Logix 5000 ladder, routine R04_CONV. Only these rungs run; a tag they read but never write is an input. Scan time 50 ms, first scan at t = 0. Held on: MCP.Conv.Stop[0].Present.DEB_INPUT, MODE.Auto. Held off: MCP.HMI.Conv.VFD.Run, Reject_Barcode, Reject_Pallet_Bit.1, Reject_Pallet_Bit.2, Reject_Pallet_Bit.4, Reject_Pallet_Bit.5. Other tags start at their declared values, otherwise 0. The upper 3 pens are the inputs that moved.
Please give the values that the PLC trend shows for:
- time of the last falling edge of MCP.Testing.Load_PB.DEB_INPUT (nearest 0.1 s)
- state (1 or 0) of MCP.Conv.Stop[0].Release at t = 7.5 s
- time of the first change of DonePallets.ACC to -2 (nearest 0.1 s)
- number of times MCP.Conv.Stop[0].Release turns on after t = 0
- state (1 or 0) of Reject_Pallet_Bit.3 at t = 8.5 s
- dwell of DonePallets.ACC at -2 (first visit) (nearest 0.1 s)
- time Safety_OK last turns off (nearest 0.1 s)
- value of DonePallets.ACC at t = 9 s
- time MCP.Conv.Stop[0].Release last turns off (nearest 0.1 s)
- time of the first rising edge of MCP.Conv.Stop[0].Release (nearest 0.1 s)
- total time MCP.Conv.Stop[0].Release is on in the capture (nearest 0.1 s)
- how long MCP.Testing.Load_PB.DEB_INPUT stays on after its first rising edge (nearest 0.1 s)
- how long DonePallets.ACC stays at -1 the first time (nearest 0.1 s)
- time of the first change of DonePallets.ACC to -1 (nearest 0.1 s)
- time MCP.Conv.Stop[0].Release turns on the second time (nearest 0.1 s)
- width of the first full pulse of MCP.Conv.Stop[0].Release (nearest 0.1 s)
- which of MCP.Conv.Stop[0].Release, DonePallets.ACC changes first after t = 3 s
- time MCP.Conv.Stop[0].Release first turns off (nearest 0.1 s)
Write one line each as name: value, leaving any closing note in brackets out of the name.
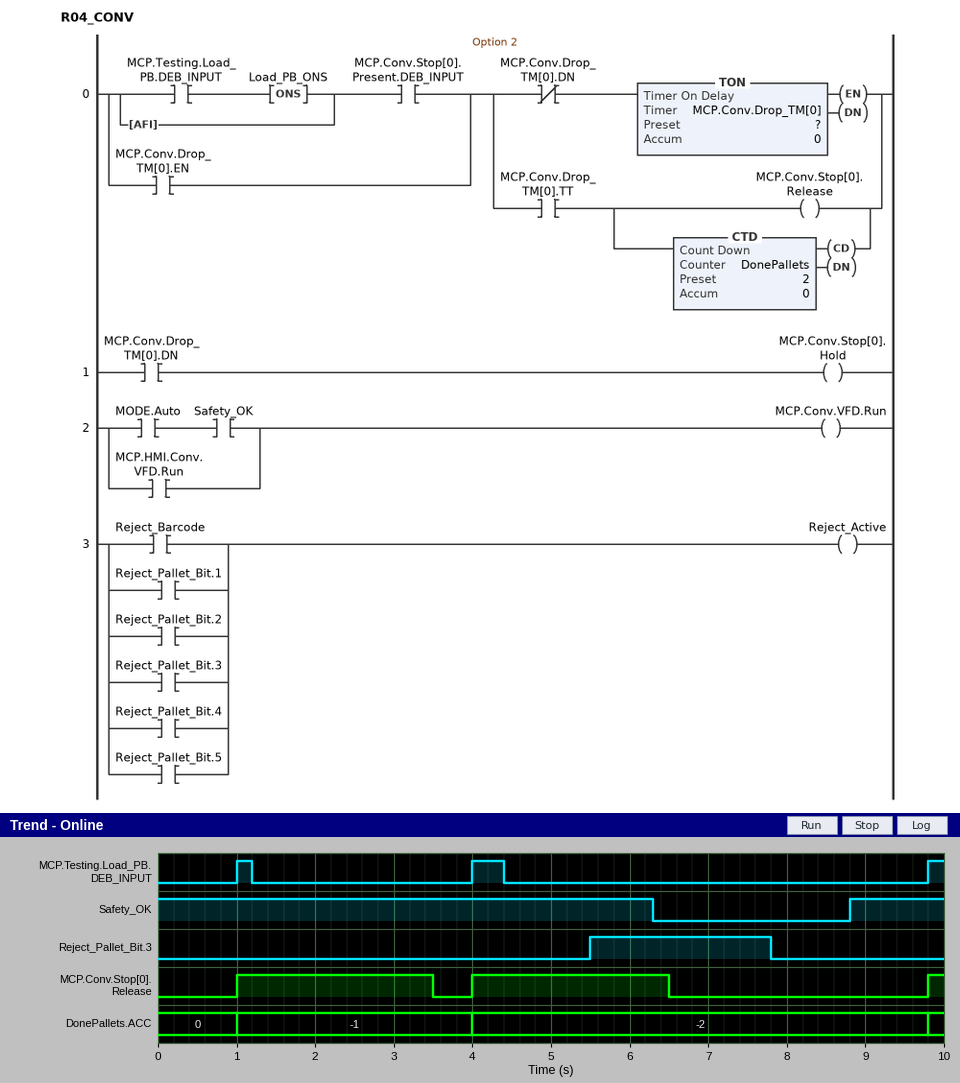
time of the last falling edge of MCP.Testing.Load_PB.DEB_INPUT: 4.4 s
state (1 or 0) of MCP.Conv.Stop[0].Release at t = 7.5 s: 0
time of the first change of DonePallets.ACC to -2: 4.0 s
number of times MCP.Conv.Stop[0].Release turns on after t = 0: 3
state (1 or 0) of Reject_Pallet_Bit.3 at t = 8.5 s: 0
dwell of DonePallets.ACC at -2 (first visit): 5.8 s
time Safety_OK last turns off: 6.3 s
value of DonePallets.ACC at t = 9 s: -2
time MCP.Conv.Stop[0].Release last turns off: 6.5 s
time of the first rising edge of MCP.Conv.Stop[0].Release: 1.0 s
total time MCP.Conv.Stop[0].Release is on in the capture: 5.2 s
how long MCP.Testing.Load_PB.DEB_INPUT stays on after its first rising edge: 0.2 s
how long DonePallets.ACC stays at -1 the first time: 3.0 s
time of the first change of DonePallets.ACC to -1: 1.0 s
time MCP.Conv.Stop[0].Release turns on the second time: 4.0 s
width of the first full pulse of MCP.Conv.Stop[0].Release: 2.5 s
which of MCP.Conv.Stop[0].Release, DonePallets.ACC changes first after t = 3 s: MCP.Conv.Stop[0].Release
time MCP.Conv.Stop[0].Release first turns off: 3.5 s
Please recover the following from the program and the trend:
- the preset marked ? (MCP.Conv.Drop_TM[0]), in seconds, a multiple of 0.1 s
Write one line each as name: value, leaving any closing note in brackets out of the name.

the preset marked ? (MCP.Conv.Drop_TM[0]), in seconds, a multiple of 0.1 s: 2.5 s
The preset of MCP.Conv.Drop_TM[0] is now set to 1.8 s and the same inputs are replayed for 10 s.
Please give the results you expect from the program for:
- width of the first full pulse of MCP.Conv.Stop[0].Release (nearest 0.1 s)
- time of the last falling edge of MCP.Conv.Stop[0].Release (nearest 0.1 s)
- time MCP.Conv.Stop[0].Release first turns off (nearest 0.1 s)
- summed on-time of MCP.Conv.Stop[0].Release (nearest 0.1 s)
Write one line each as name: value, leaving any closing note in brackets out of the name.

width of the first full pulse of MCP.Conv.Stop[0].Release: 1.8 s
time of the last falling edge of MCP.Conv.Stop[0].Release: 5.8 s
time MCP.Conv.Stop[0].Release first turns off: 2.8 s
summed on-time of MCP.Conv.Stop[0].Release: 3.8 s
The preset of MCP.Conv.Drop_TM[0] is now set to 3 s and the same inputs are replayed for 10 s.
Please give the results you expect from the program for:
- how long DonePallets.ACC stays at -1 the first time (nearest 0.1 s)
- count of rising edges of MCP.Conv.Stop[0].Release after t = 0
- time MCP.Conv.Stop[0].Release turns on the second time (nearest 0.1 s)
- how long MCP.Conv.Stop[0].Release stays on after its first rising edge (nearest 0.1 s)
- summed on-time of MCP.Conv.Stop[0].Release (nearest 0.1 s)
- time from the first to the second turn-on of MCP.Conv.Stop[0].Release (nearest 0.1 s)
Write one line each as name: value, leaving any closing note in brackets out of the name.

how long DonePallets.ACC stays at -1 the first time: 8.8 s
count of rising edges of MCP.Conv.Stop[0].Release after t = 0: 2
time MCP.Conv.Stop[0].Release turns on the second time: 9.8 s
how long MCP.Conv.Stop[0].Release stays on after its first rising edge: 3.0 s
summed on-time of MCP.Conv.Stop[0].Release: 3.2 s
time from the first to the second turn-on of MCP.Conv.Stop[0].Release: 8.8 s
